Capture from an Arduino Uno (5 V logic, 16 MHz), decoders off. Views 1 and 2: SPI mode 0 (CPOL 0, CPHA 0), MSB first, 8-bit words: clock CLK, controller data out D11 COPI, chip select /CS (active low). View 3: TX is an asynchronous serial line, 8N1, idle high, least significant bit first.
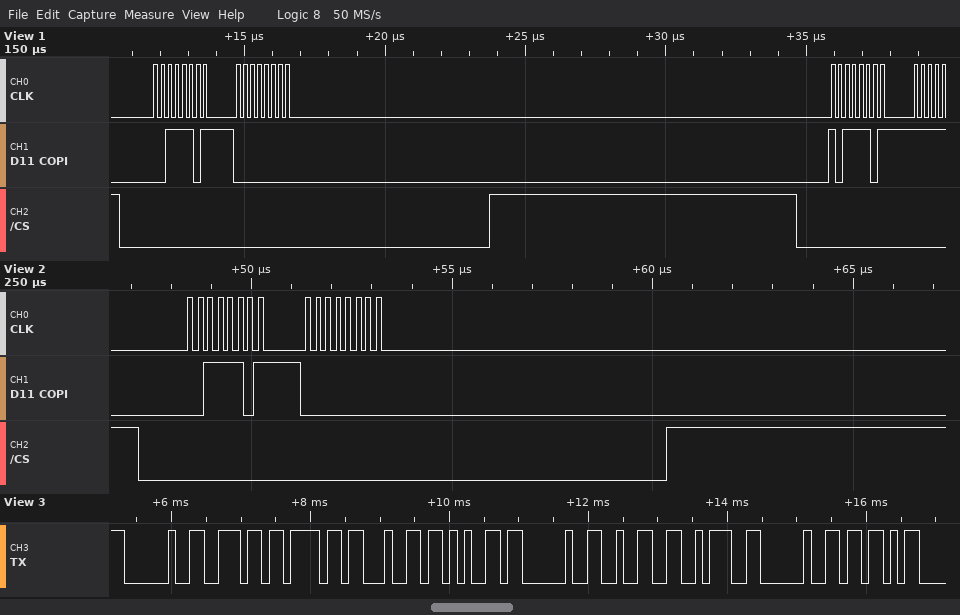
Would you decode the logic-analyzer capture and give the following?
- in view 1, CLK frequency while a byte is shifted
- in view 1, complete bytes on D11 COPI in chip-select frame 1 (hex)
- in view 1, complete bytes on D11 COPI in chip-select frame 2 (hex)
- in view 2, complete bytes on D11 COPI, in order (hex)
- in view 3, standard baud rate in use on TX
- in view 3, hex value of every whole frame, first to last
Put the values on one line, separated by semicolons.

4 MHz; 0x3D 0x00; 0xBD; 0x3D 0x00; 9600 baud; 20 6E 6F 64 65 20 32 3A 20 5B
